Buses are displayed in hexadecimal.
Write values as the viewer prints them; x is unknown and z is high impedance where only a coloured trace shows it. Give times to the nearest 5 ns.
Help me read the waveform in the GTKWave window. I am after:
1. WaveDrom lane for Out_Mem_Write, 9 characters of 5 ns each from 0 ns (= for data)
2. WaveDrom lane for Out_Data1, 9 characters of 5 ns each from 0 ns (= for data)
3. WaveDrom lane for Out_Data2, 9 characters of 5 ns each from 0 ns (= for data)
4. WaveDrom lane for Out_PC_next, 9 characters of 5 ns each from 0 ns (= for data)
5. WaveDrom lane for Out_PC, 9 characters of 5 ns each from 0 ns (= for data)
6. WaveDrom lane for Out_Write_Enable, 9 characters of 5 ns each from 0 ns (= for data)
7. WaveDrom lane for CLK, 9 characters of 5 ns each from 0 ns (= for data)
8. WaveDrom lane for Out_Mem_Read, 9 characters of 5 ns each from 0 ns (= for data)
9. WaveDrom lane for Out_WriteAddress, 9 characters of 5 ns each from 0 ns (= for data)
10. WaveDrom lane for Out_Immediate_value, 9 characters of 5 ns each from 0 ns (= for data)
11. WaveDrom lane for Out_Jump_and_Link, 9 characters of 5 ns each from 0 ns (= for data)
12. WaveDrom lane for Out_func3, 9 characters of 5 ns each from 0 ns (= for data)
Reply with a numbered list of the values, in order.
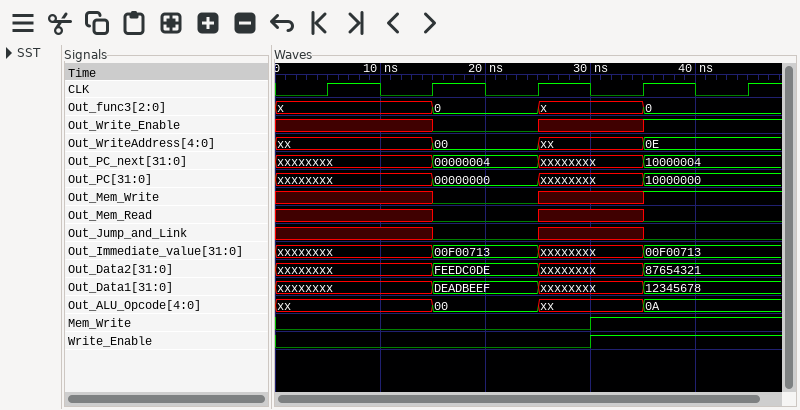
1. {name: 'Out_Mem_Write', wave: 'x..0.x.1.'}
2. {name: 'Out_Data1', wave: 'x..=.x.=.', data: 'DEADBEEF 12345678'}
3. {name: 'Out_Data2', wave: 'x..=.x.=.', data: 'FEEDC0DE 87654321'}
4. {name: 'Out_PC_next', wave: 'x..=.x.=.', data: '00000004 10000004'}
5. {name: 'Out_PC', wave: 'x..=.x.=.', data: '00000000 10000000'}
6. {name: 'Out_Write_Enable', wave: 'x..0.x.1.'}
7. {name: 'CLK', wave: '010101010'}
8. {name: 'Out_Mem_Read', wave: 'x..0.x.0.'}
9. {name: 'Out_WriteAddress', wave: 'x..=.x.=.', data: '00 0E'}
10. {name: 'Out_Immediate_value', wave: 'x..=.x.=.', data: '00F00713 00F00713'}
11. {name: 'Out_Jump_and_Link', wave: 'x..0.x.0.'}
12. {name: 'Out_func3', wave: 'x..=.x.=.', data: '0 0'}
